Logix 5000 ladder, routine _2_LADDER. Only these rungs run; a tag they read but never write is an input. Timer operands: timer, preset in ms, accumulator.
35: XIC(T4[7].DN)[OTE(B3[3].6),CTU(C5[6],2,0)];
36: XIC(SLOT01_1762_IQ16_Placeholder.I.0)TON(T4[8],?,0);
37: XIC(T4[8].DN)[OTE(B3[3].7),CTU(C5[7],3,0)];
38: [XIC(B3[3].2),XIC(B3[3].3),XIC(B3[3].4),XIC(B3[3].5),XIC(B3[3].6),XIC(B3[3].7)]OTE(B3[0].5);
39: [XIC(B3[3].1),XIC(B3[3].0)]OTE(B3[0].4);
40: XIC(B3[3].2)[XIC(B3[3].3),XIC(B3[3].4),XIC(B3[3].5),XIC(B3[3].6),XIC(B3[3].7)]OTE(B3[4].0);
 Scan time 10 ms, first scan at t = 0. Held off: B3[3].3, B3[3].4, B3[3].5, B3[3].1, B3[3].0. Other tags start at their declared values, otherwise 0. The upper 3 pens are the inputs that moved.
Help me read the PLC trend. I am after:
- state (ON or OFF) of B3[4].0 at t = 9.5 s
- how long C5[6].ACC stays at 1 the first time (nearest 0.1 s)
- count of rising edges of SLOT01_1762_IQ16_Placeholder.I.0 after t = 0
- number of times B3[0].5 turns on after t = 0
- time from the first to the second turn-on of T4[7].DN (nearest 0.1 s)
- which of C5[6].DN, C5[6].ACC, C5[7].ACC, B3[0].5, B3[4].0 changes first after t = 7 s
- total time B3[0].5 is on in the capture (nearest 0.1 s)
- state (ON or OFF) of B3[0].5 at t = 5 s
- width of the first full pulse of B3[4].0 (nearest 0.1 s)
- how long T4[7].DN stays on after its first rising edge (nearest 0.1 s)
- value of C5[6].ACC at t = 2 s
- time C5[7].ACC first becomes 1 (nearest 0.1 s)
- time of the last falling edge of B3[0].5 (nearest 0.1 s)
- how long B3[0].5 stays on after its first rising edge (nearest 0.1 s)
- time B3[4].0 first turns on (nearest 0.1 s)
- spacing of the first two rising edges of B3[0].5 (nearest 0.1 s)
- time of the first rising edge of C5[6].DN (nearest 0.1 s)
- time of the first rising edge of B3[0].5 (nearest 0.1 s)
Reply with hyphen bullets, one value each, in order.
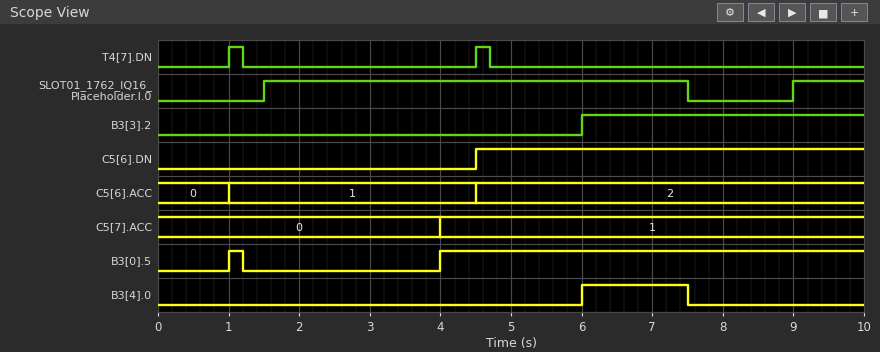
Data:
- OFF
- 3.5 s
- 2
- 2
- 3.5 s
- B3[4].0
- 6.2 s
- ON
- 1.5 s
- 0.2 s
- 1
- 4.0 s
- 1.2 s
- 0.2 s
- 6.0 s
- 3.0 s
- 4.5 s
- 1.0 s
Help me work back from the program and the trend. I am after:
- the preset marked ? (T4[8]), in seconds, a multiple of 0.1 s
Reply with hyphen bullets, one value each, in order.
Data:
- 2.5 s
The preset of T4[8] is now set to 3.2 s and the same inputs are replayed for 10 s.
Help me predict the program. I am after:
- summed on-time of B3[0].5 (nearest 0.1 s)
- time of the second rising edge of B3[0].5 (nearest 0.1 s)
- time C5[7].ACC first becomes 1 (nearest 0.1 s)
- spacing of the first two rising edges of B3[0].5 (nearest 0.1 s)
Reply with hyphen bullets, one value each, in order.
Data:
- 5.7 s
- 4.5 s
- 4.7 s
- 3.5 s
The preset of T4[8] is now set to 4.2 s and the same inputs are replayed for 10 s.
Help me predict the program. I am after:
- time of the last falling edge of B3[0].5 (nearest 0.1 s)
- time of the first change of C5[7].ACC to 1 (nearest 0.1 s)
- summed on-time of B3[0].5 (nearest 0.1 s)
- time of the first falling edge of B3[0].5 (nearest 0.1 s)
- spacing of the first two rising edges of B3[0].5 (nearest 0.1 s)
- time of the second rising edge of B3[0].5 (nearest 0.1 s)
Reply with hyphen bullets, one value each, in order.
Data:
- 4.7 s
- 5.7 s
- 4.7 s
- 1.2 s
- 3.5 s
- 4.5 s
